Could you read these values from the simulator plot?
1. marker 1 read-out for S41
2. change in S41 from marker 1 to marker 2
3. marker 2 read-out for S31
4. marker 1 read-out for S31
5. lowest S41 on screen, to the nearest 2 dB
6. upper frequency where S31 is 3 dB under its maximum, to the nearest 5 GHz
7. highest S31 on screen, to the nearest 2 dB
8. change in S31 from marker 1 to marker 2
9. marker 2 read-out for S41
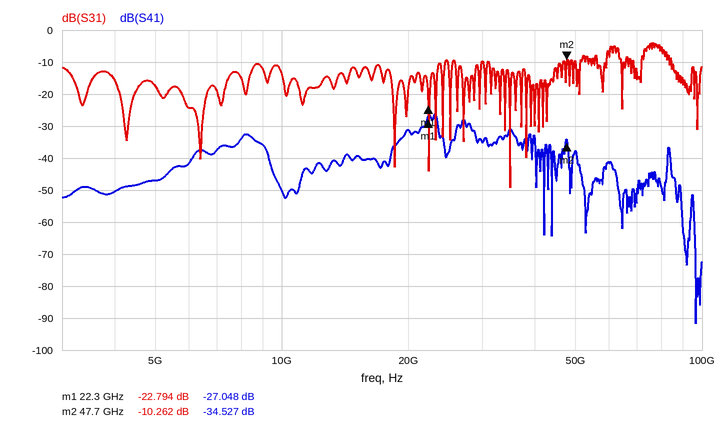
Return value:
-27.048 dB
-7.479 dB
-10.262 dB
-22.794 dB
-92 dB
80 GHz
-4 dB
12.532 dB
-34.527 dB
